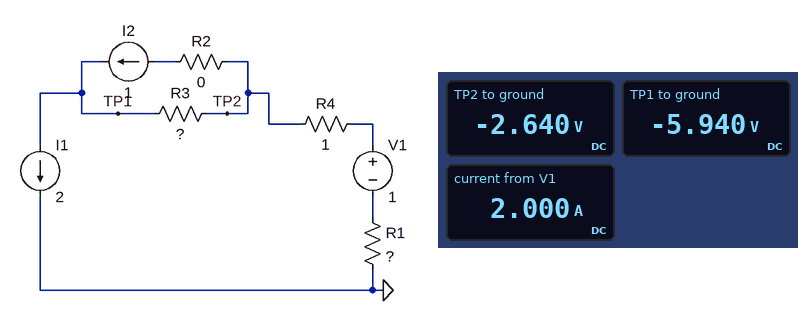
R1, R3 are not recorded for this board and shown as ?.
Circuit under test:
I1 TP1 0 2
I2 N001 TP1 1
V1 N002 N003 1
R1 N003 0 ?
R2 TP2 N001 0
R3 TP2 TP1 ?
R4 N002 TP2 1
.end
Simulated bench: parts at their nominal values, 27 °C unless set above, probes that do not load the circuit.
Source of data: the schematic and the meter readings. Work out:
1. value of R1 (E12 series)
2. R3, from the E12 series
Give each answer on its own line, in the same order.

0.82 Ω
3.3 Ω
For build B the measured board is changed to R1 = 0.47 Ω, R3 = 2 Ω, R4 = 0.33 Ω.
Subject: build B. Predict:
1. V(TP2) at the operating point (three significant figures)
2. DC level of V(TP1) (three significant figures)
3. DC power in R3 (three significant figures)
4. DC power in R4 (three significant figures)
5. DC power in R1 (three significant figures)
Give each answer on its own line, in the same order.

-600 mV
-2.60 V
2.00 W
1.32 W
1.88 W
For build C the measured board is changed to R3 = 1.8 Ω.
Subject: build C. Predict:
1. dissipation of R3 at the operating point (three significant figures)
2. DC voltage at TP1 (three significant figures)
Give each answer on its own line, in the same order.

1.80 W
-4.44 V
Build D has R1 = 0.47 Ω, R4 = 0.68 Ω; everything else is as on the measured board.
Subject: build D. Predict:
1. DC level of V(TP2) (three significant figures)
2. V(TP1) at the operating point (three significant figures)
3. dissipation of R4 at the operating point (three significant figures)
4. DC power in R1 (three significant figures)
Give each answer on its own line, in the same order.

-1.30 V
-4.60 V
2.72 W
1.88 W
